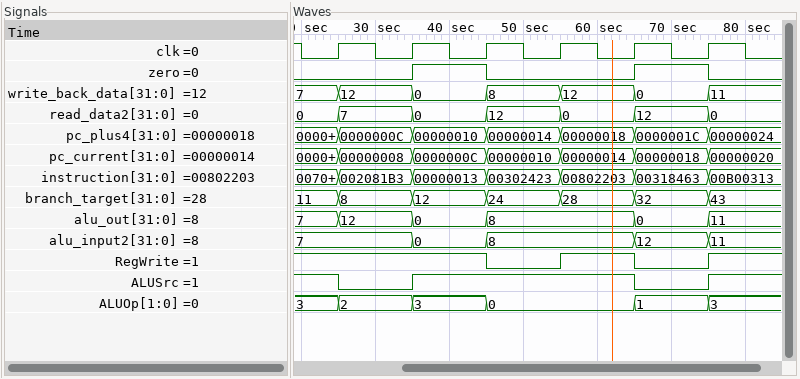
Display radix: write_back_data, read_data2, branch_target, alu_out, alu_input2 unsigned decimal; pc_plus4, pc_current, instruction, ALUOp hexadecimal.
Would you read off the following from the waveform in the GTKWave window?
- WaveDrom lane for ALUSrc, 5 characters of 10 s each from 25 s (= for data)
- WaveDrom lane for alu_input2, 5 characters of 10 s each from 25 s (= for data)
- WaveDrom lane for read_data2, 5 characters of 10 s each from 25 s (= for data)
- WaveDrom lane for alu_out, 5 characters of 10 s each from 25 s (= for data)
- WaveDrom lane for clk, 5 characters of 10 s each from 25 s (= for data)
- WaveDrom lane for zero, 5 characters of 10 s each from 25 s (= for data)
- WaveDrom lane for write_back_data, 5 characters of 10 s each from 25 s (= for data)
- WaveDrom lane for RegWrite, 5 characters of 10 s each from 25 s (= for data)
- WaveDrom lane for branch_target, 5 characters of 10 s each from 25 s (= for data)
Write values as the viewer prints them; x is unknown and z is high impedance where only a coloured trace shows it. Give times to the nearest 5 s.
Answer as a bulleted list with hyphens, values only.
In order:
- {name: 'ALUSrc', wave: '01..0'}
- {name: 'alu_input2', wave: '===.=', data: '7 0 8 12'}
- {name: 'read_data2', wave: '=====', data: '7 0 12 0 12'}
- {name: 'alu_out', wave: '===.=', data: '12 0 8 0'}
- {name: 'clk', wave: 'p....'}
- {name: 'zero', wave: '010.1'}
- {name: 'write_back_data', wave: '=====', data: '12 0 8 12 0'}
- {name: 'RegWrite', wave: '1.010'}
- {name: 'branch_target', wave: '=====', data: '8 12 24 28 32'}
